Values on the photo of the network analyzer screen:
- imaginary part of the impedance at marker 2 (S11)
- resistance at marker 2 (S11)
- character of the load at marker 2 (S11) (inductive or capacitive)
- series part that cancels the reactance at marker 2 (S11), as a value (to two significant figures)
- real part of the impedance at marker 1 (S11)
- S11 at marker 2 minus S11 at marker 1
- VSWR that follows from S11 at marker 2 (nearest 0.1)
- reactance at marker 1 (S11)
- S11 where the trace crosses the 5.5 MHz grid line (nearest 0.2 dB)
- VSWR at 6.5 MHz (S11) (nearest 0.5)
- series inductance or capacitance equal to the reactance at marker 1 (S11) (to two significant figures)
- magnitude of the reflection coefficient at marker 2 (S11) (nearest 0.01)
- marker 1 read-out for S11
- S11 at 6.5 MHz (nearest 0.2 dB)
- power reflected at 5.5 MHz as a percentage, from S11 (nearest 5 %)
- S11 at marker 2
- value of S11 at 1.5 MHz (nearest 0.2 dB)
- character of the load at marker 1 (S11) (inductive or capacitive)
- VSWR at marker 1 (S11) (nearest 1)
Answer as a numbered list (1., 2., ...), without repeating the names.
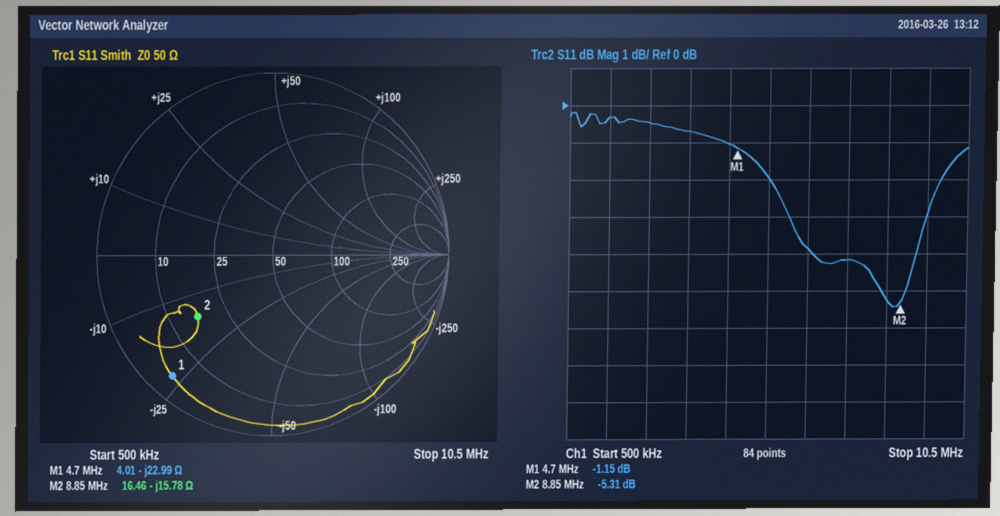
1. -15.78 Ω
2. 16.46 Ω
3. capacitive
4. 280 nH
5. 4.01 Ω
6. -4.16 dB
7. 3.4
8. -22.99 Ω
9. -2.0 dB
10. 4.5
11. 1.5 nF
12. 0.54
13. -1.15 dB
14. -3.8 dB
15. 65 %
16. -5.31 dB
17. -0.4 dB
18. capacitive
19. 15
